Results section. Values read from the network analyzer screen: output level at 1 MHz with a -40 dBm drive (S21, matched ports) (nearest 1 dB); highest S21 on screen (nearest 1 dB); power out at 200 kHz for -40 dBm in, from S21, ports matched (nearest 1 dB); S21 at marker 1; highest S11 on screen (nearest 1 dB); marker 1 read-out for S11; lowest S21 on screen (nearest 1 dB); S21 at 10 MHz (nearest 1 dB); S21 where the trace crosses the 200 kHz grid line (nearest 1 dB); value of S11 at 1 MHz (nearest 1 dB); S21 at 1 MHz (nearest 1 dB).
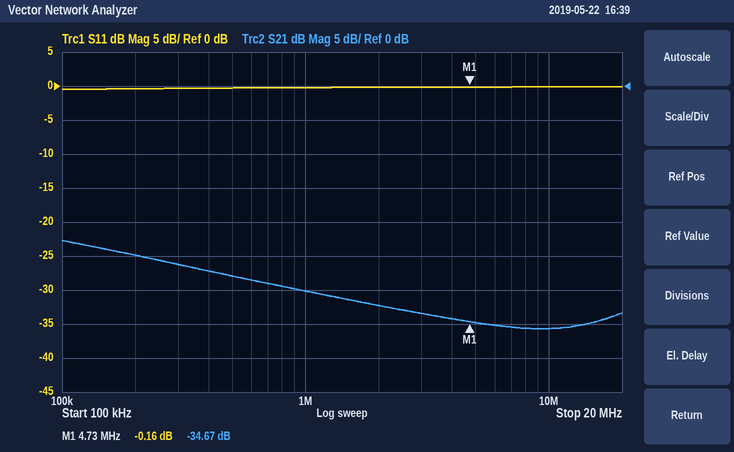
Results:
-70 dBm
-23 dB
-65 dBm
-34.67 dB
0 dB
-0.16 dB
-36 dB
-36 dB
-25 dB
0 dB
-30 dB
